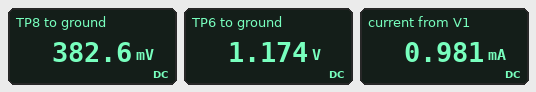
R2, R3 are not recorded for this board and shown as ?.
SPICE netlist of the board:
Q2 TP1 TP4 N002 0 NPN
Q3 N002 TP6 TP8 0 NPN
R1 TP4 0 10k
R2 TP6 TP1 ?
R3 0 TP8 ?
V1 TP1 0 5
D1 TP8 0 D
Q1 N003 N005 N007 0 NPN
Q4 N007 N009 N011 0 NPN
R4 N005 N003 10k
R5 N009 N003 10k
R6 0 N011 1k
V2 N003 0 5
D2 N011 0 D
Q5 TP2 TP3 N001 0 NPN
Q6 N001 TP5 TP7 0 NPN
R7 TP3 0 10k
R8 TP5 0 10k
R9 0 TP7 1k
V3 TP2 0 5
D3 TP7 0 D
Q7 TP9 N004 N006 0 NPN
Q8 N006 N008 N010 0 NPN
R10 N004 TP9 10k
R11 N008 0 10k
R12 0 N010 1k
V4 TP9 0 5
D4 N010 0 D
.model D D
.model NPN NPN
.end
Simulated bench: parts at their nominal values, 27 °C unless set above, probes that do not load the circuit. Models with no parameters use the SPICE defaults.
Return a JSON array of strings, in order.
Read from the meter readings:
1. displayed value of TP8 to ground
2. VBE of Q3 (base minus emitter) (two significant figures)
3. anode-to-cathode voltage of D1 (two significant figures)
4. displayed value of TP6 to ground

["382.6 mV", "790 mV", "380 mV", "1.174 V"]
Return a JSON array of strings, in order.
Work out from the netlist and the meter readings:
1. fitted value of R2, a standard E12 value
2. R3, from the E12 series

["3.9 kΩ", "390 Ω"]
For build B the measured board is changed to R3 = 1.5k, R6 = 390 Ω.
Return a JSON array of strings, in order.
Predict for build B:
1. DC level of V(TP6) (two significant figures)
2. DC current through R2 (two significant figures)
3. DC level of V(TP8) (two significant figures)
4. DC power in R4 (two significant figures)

["1.4 V", "920 µA", "640 mV", "1.0 mW"]
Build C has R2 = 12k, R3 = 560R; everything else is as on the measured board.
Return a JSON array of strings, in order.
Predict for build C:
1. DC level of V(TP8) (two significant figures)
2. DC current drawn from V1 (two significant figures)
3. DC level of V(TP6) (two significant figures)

["190 mV", "340 µA", "950 mV"]
